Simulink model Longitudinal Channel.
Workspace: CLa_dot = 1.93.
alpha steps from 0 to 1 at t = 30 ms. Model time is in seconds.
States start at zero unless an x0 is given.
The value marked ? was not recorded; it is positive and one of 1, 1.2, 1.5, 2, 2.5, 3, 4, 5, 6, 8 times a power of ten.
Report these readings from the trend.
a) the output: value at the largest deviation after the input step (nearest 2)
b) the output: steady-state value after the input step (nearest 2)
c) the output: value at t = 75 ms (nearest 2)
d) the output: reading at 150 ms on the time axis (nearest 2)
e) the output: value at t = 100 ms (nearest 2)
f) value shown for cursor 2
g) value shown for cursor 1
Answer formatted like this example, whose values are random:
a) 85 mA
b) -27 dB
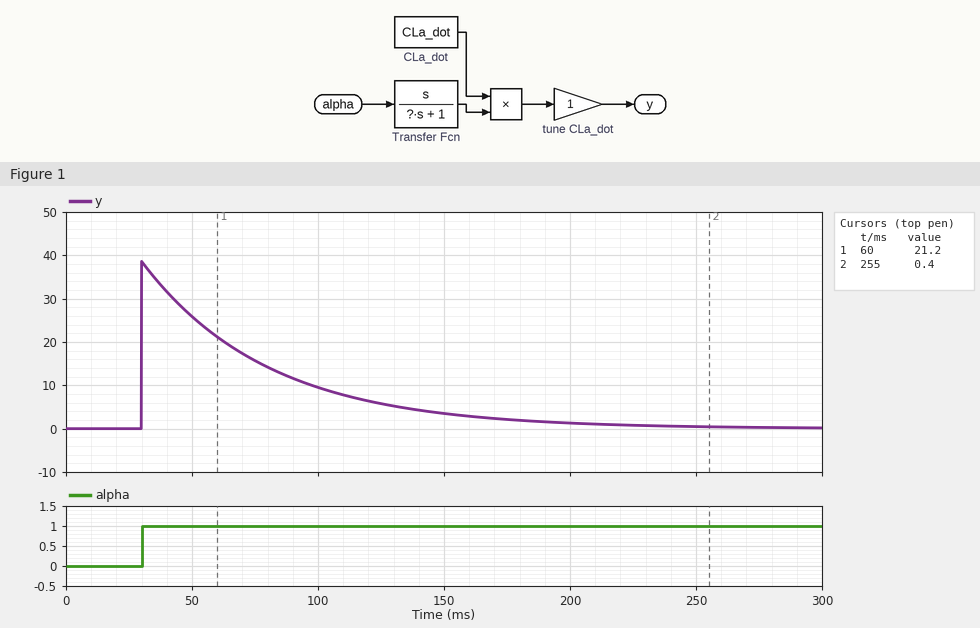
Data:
a) 38
b) 0
c) 16
d) 4
e) 10
f) 0.4
g) 21.2
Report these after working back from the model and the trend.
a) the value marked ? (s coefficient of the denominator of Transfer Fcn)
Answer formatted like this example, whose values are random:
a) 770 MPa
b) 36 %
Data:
a) 0.05
